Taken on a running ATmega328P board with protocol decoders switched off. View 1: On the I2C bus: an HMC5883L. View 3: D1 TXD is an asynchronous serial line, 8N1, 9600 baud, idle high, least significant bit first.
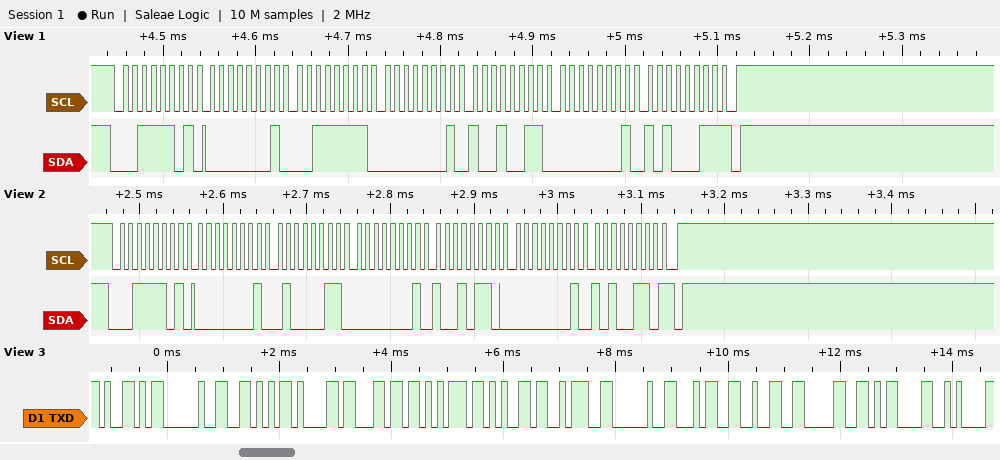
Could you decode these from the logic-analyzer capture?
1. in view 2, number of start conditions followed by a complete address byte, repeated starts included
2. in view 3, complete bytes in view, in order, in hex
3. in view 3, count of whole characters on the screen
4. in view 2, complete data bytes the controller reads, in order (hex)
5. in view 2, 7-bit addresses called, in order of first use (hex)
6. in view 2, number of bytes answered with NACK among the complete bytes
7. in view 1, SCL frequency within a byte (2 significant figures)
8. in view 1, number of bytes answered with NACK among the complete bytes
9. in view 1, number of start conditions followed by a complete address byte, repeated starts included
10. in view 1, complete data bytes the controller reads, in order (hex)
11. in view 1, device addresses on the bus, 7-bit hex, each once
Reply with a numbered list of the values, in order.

1. 1
2. 59 20 56 61 6C 75 65 3A 20 34 32 30 0D 0A
3. 14
4. 01 43 01 96 01 A6
5. 0x1E
6. 1
7. 100 kHz
8. 1
9. 1
10. 01 3F 01 93 01 A3
11. 0x1E
